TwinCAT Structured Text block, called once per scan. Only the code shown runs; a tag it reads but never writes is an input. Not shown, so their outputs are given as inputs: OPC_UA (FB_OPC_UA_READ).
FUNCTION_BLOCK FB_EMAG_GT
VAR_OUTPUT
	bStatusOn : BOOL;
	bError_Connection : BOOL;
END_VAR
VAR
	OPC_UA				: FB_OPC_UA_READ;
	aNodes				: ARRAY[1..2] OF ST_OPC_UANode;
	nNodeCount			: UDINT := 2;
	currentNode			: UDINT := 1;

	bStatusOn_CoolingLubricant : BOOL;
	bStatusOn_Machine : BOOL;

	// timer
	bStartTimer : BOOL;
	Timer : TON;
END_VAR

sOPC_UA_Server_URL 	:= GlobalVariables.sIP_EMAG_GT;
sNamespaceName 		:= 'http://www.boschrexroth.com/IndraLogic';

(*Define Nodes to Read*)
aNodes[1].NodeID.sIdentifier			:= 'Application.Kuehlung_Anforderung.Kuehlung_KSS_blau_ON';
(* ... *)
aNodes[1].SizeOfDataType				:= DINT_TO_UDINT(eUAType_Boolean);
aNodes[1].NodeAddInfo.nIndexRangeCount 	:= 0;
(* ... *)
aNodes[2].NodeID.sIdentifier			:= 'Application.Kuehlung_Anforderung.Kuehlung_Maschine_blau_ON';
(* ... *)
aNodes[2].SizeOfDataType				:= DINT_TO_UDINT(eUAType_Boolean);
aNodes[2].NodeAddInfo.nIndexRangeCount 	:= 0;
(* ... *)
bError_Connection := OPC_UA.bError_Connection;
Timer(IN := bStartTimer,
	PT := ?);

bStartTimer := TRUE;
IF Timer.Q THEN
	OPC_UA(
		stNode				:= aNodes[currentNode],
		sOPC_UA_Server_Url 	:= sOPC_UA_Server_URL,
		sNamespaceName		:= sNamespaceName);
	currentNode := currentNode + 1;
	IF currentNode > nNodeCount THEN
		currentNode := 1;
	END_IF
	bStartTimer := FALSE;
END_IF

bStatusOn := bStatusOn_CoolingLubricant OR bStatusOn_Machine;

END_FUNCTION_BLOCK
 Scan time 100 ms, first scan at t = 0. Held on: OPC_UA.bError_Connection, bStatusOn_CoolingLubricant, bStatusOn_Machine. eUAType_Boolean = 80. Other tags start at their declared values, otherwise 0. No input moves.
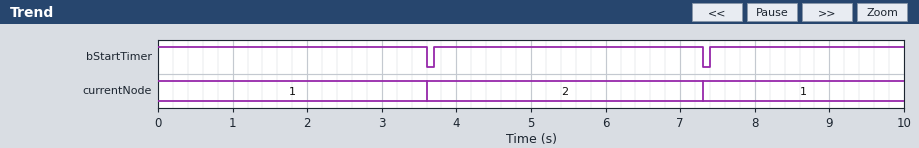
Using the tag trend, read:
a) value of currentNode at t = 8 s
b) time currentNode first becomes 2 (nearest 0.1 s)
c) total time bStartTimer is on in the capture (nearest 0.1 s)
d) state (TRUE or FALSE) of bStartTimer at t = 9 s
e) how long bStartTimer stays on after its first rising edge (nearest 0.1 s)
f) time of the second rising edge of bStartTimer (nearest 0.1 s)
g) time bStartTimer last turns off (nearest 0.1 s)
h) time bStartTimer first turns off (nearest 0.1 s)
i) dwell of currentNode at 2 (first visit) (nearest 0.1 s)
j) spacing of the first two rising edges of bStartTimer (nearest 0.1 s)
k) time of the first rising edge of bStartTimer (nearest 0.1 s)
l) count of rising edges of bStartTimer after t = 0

1
3.6 s
9.8 s
TRUE
3.6 s
7.4 s
7.3 s
3.6 s
3.7 s
3.7 s
3.7 s
2
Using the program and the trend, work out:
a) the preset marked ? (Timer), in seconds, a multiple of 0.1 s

3.5 s
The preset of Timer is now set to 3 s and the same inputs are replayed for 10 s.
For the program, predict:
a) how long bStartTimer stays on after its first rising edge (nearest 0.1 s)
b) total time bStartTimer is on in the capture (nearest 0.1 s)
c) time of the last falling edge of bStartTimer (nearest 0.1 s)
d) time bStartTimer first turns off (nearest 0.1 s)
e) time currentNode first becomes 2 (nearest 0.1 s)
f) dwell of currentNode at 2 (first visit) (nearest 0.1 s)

3.1 s
9.7 s
9.5 s
3.1 s
3.1 s
3.2 s
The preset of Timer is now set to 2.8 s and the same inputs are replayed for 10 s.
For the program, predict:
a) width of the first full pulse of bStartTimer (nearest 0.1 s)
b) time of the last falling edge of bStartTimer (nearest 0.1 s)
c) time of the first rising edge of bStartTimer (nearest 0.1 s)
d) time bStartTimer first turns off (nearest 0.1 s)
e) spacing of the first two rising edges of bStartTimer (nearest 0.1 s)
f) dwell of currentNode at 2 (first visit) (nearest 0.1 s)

2.9 s
8.9 s
3.0 s
2.9 s
3.0 s
3.0 s
